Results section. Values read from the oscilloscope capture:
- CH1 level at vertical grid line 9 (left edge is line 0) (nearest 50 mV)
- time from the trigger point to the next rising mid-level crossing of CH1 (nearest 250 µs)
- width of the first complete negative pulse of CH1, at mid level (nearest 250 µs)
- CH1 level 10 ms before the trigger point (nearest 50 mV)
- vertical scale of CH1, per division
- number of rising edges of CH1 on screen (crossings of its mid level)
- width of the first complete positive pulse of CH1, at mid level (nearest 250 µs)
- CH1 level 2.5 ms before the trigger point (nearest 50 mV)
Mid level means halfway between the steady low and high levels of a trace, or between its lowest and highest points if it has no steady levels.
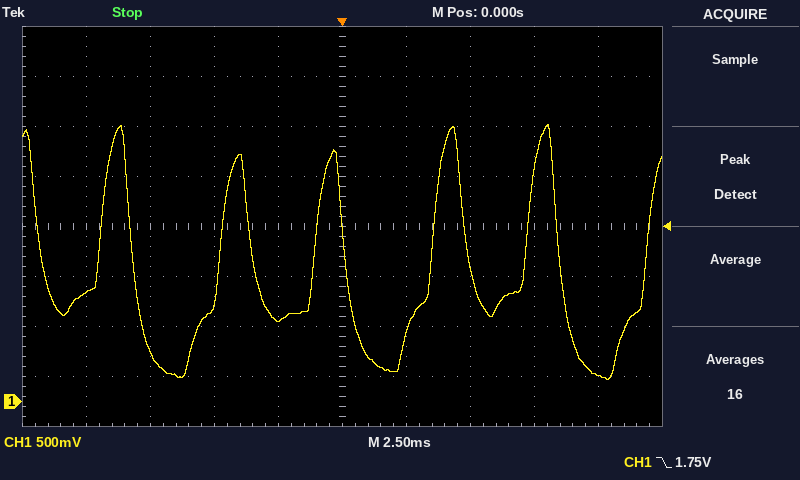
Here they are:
250 mV
3.50 ms
2.25 ms
1.10 V
500 mV
6
1.25 ms
800 mV
